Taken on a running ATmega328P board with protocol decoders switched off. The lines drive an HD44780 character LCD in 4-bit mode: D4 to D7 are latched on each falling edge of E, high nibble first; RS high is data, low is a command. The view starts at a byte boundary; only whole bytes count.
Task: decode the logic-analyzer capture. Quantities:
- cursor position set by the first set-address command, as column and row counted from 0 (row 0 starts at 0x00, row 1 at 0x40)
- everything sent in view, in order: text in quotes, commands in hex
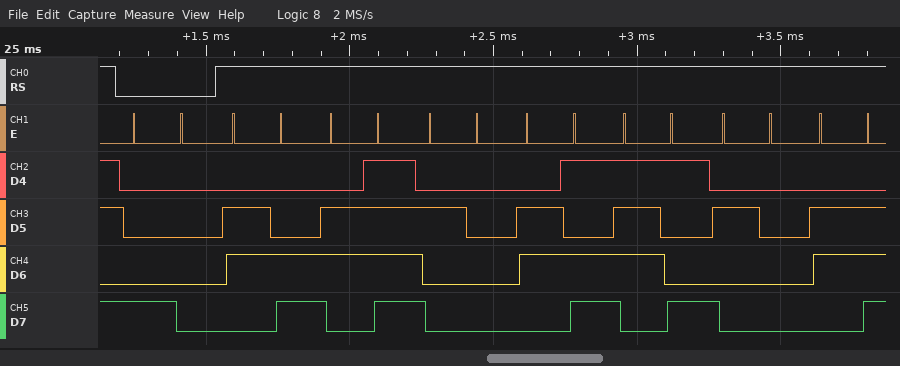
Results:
column 0, row 0
0x80 "lo my n"
